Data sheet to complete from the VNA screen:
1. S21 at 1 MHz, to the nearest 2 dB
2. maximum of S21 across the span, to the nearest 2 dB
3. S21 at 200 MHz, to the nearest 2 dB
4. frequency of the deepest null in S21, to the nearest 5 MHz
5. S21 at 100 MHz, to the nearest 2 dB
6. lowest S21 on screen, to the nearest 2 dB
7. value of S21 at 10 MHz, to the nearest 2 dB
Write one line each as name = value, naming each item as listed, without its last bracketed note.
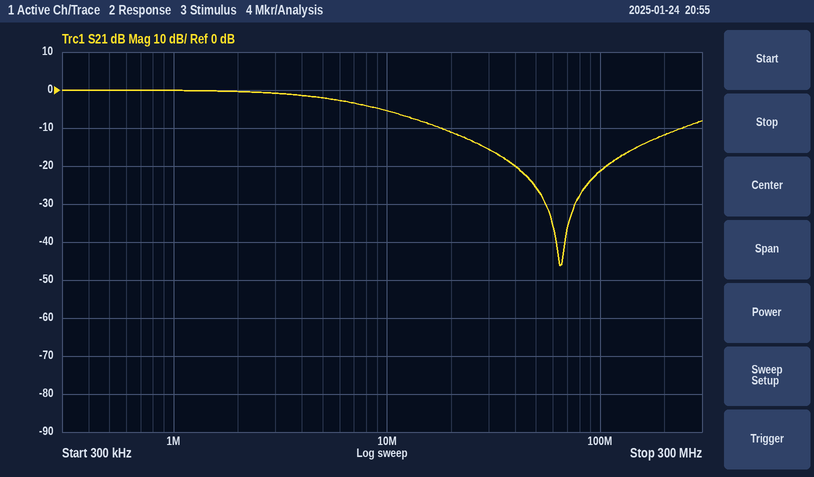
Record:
S21 at 1 MHz, to the nearest 2 dB = 0 dB
maximum of S21 across the span, to the nearest 2 dB = 0 dB
S21 at 200 MHz, to the nearest 2 dB = -12 dB
frequency of the deepest null in S21, to the nearest 5 MHz = 65 MHz
S21 at 100 MHz, to the nearest 2 dB = -22 dB
lowest S21 on screen, to the nearest 2 dB = -46 dB
value of S21 at 10 MHz, to the nearest 2 dB = -6 dB
